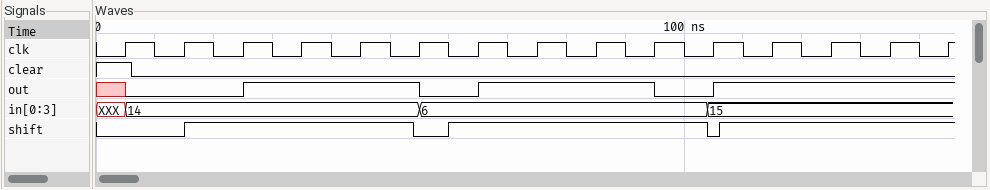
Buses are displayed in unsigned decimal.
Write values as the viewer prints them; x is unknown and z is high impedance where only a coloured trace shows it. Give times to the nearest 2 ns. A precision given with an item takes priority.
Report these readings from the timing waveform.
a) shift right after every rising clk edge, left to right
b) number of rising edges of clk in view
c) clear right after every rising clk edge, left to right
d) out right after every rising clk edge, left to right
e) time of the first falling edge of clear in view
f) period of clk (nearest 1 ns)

0 1 1 1 1 0 1 1 1 1 0 1 1 1 1
15
1 0 0 0 0 0 0 0 0 0 0 0 0 0 0
0 0 1 1 1 0 1 1 1 0 1 1 1 1 1
6 ns
10 ns
